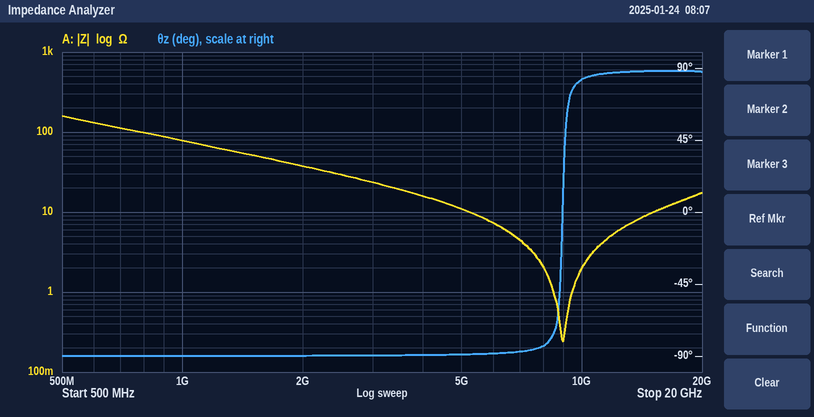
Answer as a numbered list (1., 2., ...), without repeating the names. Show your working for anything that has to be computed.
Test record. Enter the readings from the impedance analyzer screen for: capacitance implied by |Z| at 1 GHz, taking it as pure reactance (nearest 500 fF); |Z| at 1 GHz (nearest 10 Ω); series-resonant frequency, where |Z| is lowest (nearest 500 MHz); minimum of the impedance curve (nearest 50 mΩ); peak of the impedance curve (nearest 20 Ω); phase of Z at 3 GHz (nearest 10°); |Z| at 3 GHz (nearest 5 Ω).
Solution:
1. C = 1/(2π × 1 GHz × 80 Ω) ≈ 2.0 pF
2. 80 Ω
3. 9.0 GHz
4. 250 mΩ
5. 160 Ω
6. -90°
7. 25 Ω
